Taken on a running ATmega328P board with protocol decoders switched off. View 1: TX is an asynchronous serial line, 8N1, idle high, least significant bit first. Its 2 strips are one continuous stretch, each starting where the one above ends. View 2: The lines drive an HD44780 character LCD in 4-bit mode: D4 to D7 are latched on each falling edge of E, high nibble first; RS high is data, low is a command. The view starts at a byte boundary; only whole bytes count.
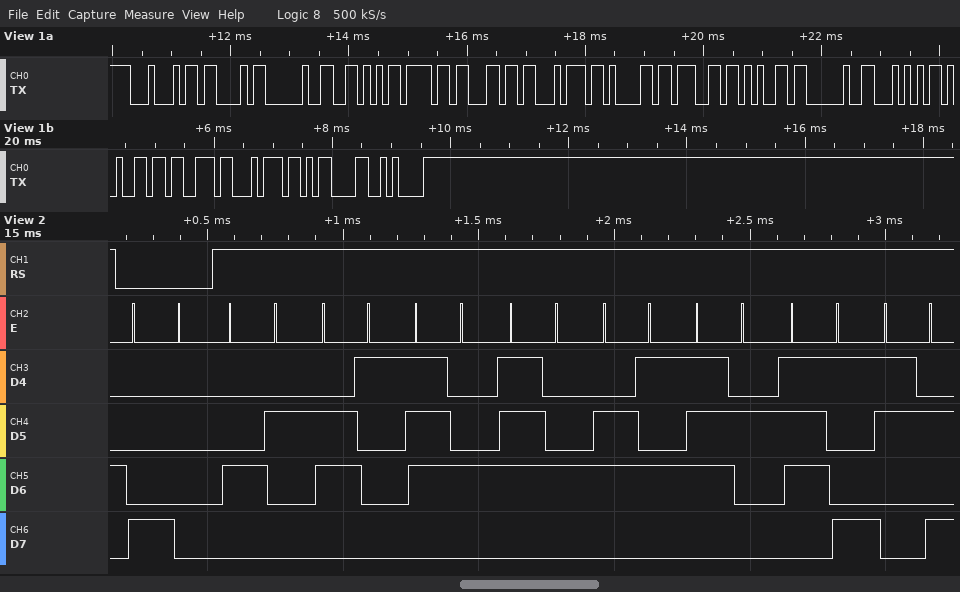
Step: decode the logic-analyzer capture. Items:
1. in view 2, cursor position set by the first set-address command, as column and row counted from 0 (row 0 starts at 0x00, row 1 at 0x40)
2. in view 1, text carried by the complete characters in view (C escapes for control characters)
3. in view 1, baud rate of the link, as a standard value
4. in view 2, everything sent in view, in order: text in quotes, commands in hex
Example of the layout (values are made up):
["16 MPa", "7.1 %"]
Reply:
["column 0, row 0", "\"DC Voltage Test\\r\\n\"", "9600 baud", "0x80 \"Battery:\""]
